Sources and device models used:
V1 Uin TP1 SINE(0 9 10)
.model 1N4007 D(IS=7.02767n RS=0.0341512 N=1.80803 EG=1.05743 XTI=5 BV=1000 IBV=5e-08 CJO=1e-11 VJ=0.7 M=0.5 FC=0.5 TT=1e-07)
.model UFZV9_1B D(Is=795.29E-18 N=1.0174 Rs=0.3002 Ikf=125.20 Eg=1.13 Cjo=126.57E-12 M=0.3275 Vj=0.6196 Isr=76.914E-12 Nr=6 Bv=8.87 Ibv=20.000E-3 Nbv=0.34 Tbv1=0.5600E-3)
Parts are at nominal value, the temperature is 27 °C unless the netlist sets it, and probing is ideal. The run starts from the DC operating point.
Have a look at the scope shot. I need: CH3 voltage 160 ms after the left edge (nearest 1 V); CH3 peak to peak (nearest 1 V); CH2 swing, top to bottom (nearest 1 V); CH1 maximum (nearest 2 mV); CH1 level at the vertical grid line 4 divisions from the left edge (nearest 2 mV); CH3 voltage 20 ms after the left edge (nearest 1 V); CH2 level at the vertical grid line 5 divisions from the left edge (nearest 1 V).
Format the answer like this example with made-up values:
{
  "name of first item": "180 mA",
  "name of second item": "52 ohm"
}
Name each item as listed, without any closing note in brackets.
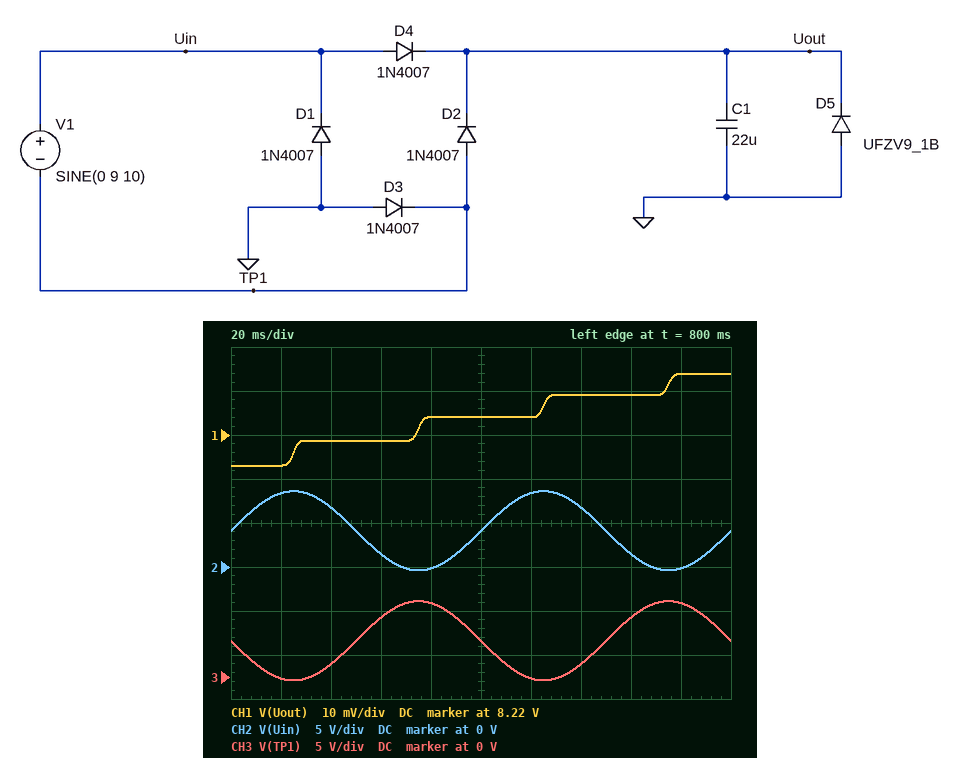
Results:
{
  "CH3 voltage 160 ms after the left edge": "7 V",
  "CH3 peak to peak": "9 V",
  "CH2 swing, top to bottom": "9 V",
  "CH1 maximum": "8.234 V",
  "CH1 level at the vertical grid line 4 divisions from the left edge": "8.224 V",
  "CH3 voltage 20 ms after the left edge": "0 V",
  "CH2 level at the vertical grid line 5 divisions from the left edge": "4 V"
}
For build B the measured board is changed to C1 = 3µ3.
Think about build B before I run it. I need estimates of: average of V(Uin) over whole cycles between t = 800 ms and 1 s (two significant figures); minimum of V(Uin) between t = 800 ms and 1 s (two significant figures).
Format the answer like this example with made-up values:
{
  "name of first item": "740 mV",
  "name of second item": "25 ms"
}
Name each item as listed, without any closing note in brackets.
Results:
{
  "average of V(Uin) over whole cycles between t = 800 ms and 1 s": "4.2 V",
  "minimum of V(Uin) between t = 800 ms and 1 s": "-300 mV"
}
